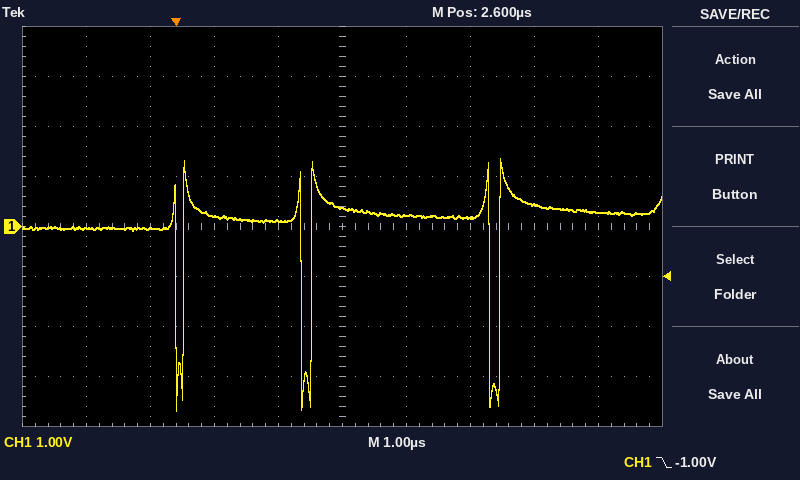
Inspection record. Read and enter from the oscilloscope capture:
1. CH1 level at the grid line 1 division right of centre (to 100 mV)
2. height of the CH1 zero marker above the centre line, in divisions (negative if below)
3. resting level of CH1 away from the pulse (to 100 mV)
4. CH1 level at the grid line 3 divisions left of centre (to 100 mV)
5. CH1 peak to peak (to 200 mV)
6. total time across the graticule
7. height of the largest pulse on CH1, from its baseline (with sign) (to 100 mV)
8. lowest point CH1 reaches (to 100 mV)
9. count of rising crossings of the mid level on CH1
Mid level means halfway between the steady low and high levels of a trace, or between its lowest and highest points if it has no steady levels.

200 mV
0.0 div
200 mV
0.0 V
5.0 V
10 µs
-3.9 V
-3.7 V
3
